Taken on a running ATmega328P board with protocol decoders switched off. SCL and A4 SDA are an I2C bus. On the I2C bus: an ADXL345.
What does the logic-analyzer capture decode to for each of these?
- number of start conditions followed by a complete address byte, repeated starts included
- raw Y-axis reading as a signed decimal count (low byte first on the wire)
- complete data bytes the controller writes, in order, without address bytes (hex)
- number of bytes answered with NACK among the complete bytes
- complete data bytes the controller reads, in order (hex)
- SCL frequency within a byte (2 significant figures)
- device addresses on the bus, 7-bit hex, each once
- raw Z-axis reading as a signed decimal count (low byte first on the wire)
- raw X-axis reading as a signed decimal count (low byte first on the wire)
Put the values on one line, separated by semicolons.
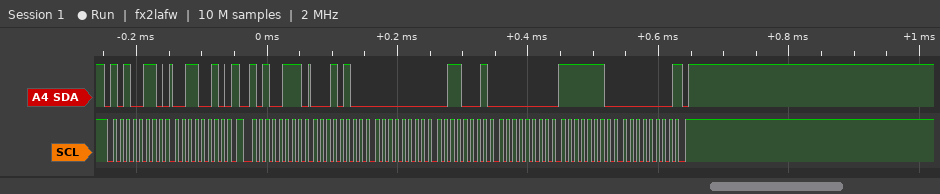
2; 49; 32; 1; 14 00 31 00 FE 00; 100 kHz; 0x53; 254; 20
